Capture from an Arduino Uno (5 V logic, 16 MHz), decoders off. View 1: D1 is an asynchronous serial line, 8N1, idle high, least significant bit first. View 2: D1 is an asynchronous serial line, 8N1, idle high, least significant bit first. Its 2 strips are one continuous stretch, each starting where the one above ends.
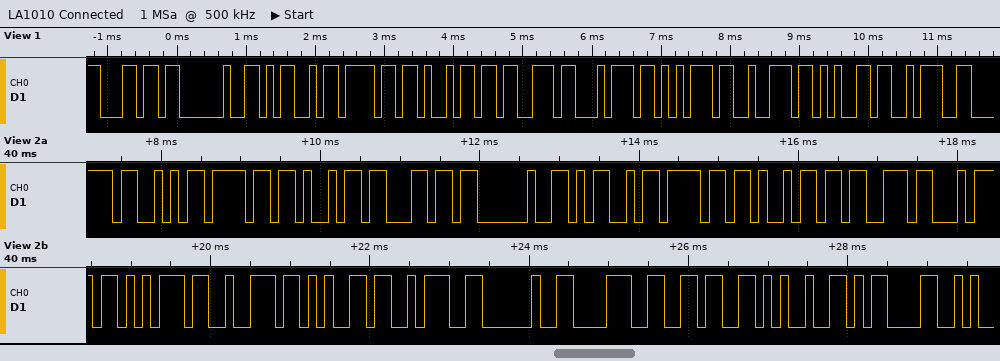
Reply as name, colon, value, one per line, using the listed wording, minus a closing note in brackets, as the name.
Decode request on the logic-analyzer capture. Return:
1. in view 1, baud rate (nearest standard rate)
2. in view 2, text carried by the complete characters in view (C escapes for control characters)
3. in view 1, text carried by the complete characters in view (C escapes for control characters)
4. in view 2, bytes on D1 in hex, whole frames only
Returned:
in view 1, baud rate: 9600 baud
in view 2, text carried by the complete characters in view: "Soil Moisture: 86%\r"
in view 1, text carried by the complete characters in view: "l Moisture:"
in view 2, bytes on D1 in hex, whole frames only: 53 6F 69 6C 20 4D 6F 69 73 74 75 72 65 3A 20 38 36 25 0D
